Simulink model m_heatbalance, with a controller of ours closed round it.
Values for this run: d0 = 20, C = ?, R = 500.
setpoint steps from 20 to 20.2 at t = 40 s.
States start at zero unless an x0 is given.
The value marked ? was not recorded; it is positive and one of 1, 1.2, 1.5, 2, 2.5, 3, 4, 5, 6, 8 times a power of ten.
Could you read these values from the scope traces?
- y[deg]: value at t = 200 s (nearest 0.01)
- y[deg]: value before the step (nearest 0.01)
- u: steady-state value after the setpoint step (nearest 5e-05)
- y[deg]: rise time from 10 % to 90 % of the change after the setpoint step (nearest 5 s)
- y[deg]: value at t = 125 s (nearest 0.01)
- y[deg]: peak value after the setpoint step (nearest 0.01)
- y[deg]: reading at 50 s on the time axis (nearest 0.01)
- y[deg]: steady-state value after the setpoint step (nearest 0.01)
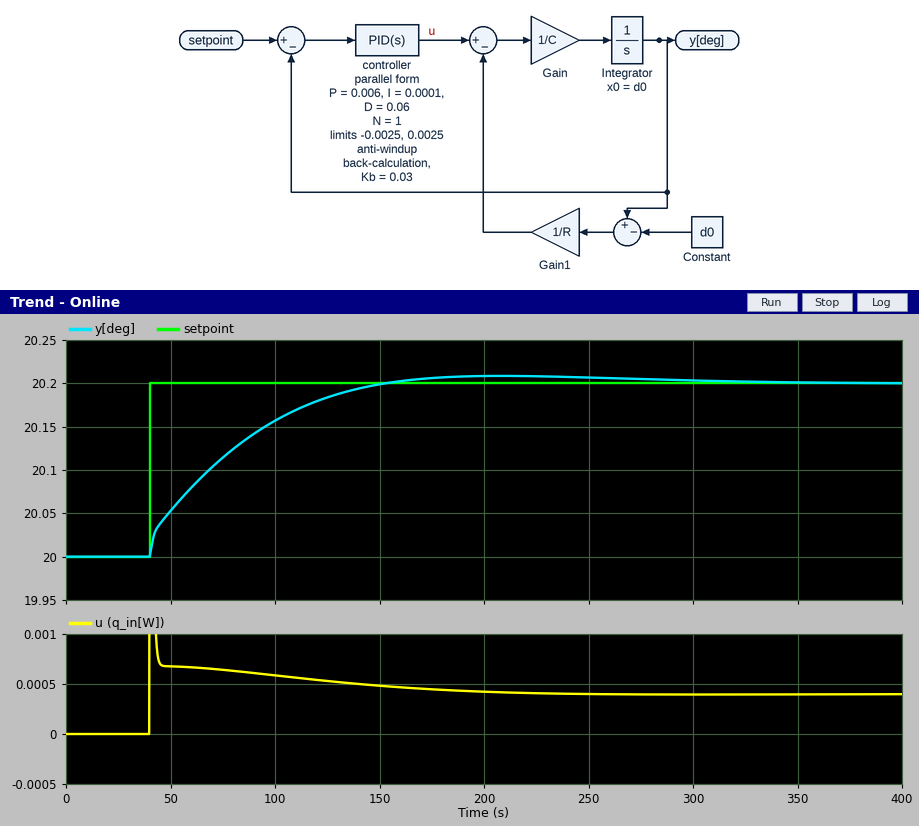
20.21
20.00
0.00040
80 s
20.18
20.21
20.05
20.20
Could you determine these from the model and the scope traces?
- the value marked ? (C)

0.2
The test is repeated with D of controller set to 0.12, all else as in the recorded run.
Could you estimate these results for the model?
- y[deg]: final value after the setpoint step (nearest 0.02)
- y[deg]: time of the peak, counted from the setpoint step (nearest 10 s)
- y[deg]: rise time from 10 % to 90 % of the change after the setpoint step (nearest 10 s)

20.20
210 s
110 s
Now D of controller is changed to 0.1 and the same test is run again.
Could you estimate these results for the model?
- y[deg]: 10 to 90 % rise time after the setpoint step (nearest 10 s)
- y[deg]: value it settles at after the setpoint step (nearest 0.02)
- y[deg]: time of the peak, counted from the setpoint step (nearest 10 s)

100 s
20.20
200 s
